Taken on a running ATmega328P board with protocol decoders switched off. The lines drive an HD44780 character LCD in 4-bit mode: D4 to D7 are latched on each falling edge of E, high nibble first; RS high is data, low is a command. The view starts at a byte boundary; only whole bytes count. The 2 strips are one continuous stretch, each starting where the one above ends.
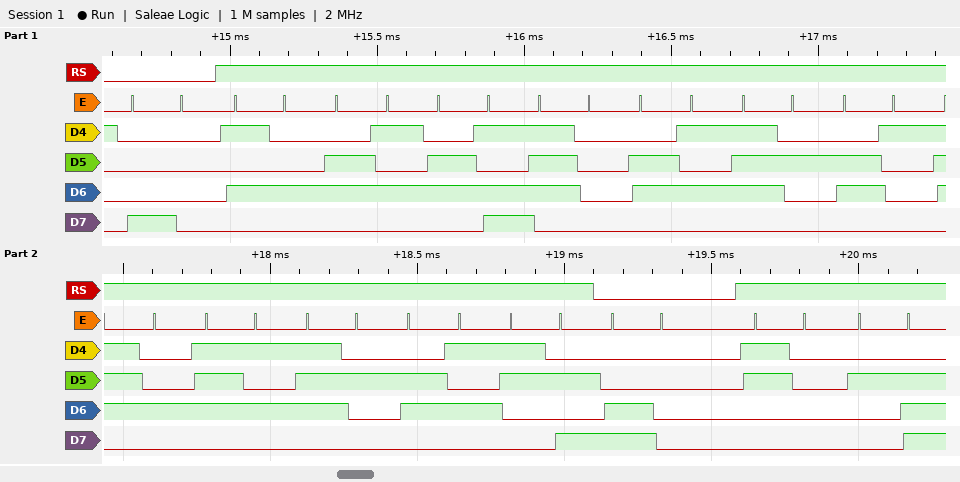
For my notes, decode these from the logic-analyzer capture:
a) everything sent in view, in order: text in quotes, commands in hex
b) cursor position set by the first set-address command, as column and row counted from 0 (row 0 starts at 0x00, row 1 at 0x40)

0x80 "Temperature:" 0xC0 "0."
column 0, row 0
